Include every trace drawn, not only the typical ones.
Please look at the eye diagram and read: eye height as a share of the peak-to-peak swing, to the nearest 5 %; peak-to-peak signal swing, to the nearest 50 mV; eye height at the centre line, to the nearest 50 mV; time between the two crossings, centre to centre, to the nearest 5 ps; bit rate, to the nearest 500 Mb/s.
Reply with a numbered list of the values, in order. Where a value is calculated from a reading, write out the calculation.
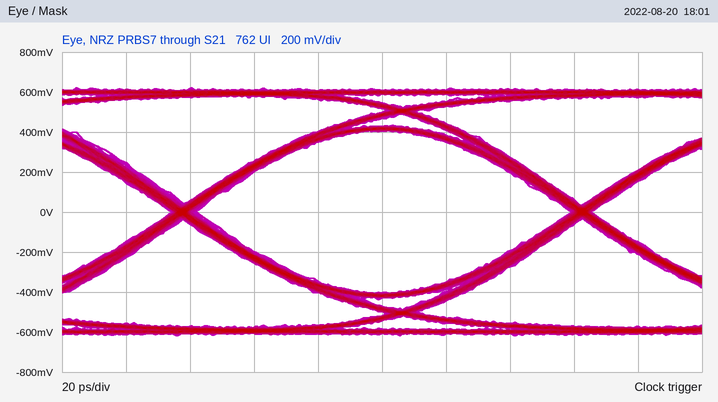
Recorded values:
1. 800 mV / 1.25 V ≈ 64.0 %, so 65 % to the nearest 5 %
2. 1.25 V
3. 800 mV
4. 125 ps
5. 8.0 Gb/s
